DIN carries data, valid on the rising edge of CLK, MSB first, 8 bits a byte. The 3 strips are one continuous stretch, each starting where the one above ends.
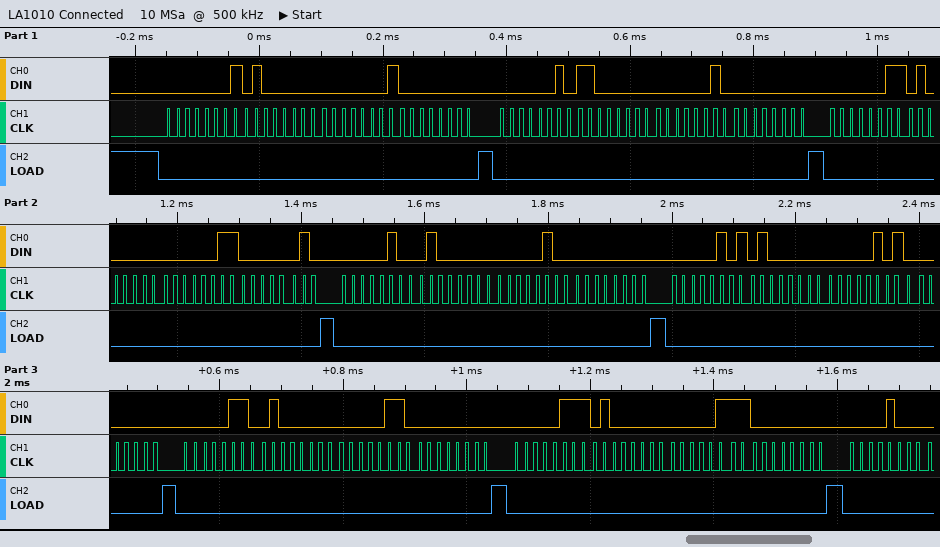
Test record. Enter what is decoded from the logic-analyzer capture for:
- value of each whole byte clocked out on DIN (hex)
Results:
01 40 01 00 02 C0 02 00 03 40 03 02 04 40 04 00 05 40 05 00 06 40 06 00 07 40 07 00 08
